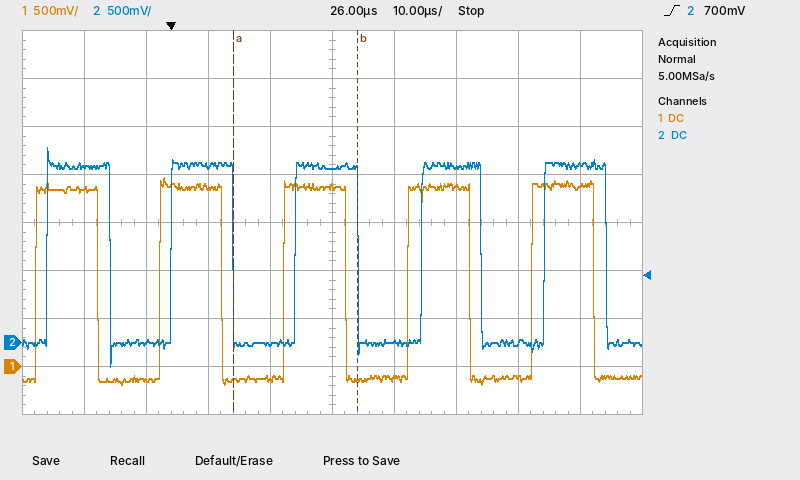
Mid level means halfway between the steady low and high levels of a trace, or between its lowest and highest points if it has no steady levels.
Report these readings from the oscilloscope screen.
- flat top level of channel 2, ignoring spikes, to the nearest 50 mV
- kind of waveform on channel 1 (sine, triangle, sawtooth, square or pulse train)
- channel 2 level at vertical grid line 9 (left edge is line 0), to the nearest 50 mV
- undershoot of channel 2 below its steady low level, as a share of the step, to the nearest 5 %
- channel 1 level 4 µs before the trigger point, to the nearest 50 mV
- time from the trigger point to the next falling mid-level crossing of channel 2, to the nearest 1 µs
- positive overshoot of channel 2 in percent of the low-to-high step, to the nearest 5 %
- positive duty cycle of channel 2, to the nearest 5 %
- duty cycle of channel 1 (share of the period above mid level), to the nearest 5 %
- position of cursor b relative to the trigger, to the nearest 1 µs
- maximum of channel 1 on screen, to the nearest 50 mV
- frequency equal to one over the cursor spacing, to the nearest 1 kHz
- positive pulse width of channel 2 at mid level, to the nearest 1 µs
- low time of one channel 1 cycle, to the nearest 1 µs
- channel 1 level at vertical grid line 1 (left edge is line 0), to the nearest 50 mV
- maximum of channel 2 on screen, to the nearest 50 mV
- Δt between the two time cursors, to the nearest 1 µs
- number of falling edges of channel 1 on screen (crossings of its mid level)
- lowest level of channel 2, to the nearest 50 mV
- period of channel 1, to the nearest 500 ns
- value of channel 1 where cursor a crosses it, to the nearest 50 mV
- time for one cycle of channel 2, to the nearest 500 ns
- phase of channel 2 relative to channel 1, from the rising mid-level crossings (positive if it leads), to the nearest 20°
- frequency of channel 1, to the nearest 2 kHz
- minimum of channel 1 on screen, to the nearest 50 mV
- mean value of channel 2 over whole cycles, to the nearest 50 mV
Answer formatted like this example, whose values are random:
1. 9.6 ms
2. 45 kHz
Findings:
1. 1.85 V
2. square
3. 1.85 V
4. 15 %
5. -150 mV
6. 10 µs
7. 10 %
8. 50 %
9. 50 %
10. +30 µs
11. 1.95 V
12. 50 kHz
13. 10 µs
14. 10 µs
15. 1.85 V
16. 2.05 V
17. 20 µs
18. 5
19. -250 mV
20. 20.0 µs
21. -150 mV
22. 20.0 µs
23. -40°
24. 50 kHz
25. -200 mV
26. 900 mV
